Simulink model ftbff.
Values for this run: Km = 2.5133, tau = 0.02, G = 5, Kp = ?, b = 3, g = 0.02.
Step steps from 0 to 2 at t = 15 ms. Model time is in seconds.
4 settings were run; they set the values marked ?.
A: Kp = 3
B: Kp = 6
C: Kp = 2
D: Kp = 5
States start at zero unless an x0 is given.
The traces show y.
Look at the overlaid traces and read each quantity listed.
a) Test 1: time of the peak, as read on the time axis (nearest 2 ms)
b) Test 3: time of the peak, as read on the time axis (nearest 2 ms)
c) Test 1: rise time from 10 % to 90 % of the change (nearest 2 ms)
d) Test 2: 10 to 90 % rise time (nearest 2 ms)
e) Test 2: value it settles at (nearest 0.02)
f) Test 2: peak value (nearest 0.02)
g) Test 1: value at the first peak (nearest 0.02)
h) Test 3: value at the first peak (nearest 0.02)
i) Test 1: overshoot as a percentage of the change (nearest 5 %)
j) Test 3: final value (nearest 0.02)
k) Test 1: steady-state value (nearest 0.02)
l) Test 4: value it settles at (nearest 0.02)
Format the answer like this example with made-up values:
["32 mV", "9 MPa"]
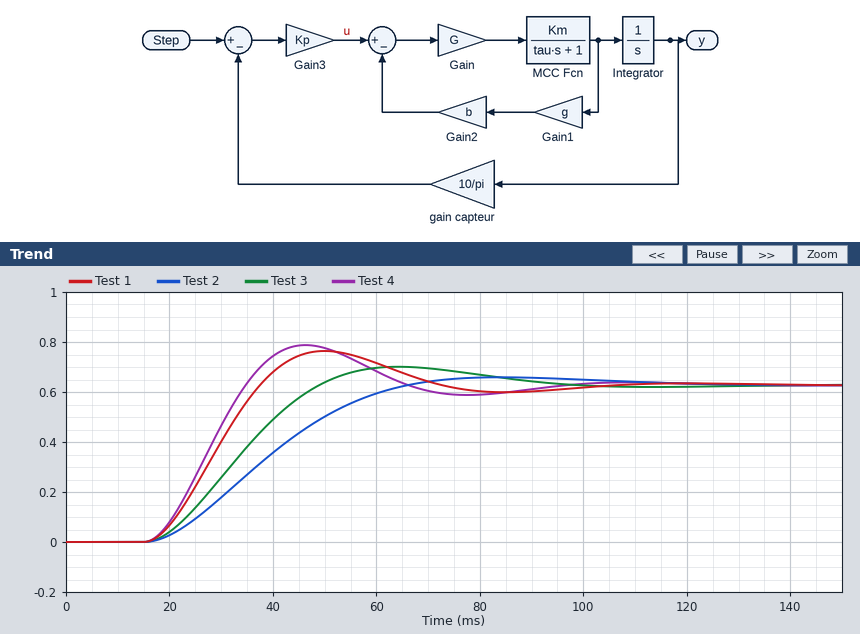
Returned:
["50 ms", "64 ms", "16 ms", "34 ms", "0.62", "0.66", "0.76", "0.70", "20 %", "0.62", "0.62", "0.62"]
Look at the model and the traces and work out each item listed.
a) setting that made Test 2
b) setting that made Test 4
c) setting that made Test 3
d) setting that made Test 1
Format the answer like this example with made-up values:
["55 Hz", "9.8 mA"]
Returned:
["C", "B", "A", "D"]
